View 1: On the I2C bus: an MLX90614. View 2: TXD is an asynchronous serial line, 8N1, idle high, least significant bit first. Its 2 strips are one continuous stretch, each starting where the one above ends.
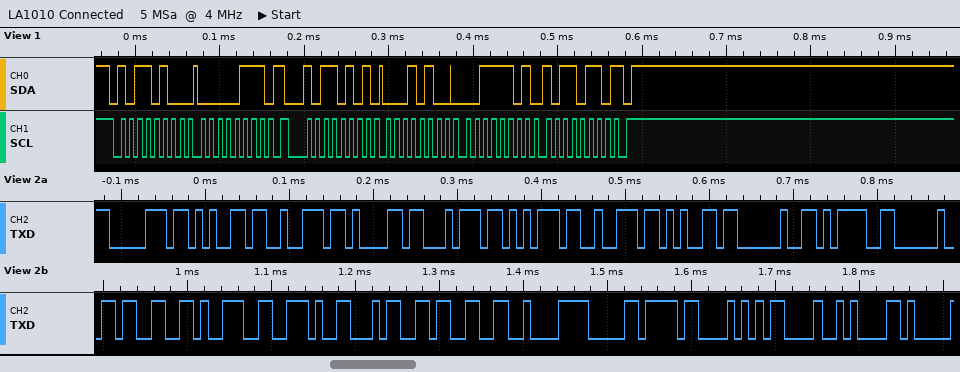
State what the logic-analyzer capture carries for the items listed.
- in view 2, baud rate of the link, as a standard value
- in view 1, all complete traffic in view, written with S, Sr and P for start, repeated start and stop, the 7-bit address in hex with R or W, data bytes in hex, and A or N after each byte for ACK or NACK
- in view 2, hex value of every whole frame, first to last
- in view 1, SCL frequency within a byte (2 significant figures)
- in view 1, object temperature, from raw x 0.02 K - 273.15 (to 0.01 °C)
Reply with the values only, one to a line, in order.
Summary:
115200 baud
S 5AW A 07 A Sr 5AR A 14 A 3D A B6 N P
70 65 72 61 74 75 72 65 20 3D 20 33 39 2E 34 33 C2 B0 43 0D 0A
100 kHz
39.57 °C
